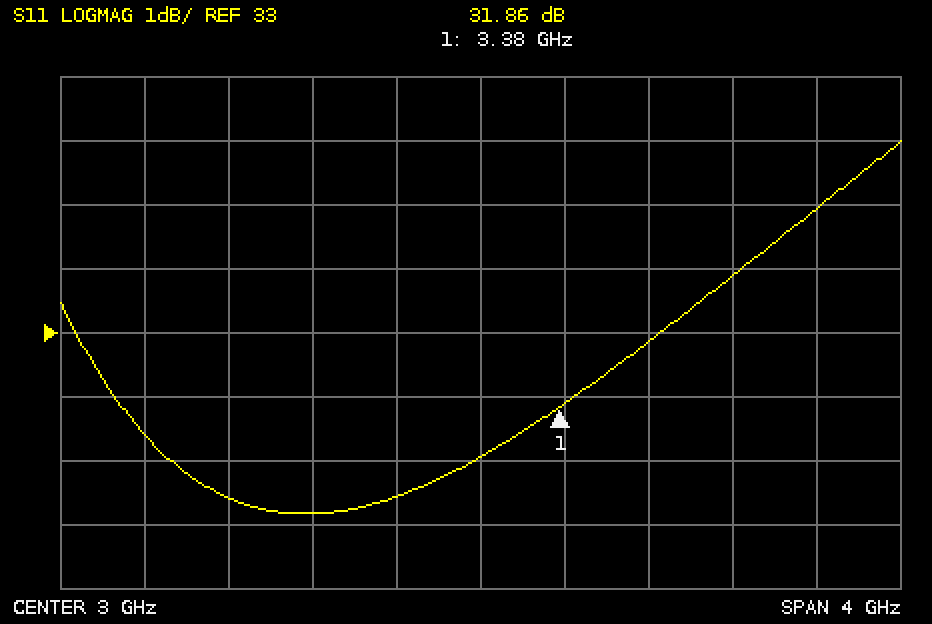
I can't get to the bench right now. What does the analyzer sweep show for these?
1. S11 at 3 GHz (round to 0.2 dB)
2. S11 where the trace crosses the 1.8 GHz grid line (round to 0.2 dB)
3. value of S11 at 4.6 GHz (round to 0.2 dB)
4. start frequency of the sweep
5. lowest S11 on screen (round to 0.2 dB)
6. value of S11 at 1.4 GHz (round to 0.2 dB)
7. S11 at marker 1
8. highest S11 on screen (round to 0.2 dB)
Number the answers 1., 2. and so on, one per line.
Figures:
1. 31.0 dB
2. 30.4 dB
3. 35.0 dB
4. 1 GHz
5. 30.2 dB
6. 31.4 dB
7. 31.86 dB
8. 36.0 dB
